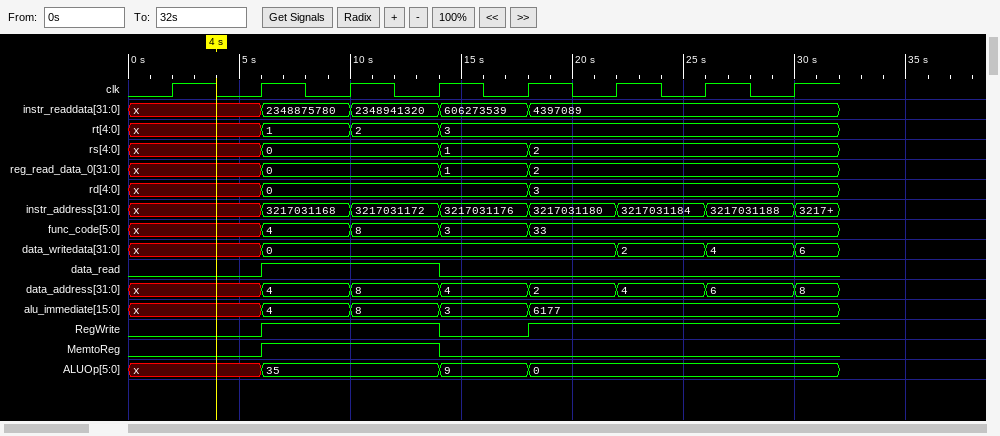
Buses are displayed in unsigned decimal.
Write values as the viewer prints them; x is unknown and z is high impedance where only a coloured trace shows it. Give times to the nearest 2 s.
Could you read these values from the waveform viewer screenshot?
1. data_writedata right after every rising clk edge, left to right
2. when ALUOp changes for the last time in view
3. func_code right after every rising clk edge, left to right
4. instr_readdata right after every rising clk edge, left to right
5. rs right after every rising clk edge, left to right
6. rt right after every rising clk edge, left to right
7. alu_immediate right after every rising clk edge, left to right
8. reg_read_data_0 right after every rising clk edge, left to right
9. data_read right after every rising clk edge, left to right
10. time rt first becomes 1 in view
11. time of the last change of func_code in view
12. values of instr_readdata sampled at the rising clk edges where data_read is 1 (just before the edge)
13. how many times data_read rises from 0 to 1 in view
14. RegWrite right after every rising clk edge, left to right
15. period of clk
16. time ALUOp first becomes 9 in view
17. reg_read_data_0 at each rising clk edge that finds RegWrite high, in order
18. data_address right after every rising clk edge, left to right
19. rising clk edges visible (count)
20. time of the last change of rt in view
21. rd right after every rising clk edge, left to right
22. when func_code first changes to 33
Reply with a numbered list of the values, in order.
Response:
1. x, 0, 0, 0, 0, 2, 4, 6
2. 18 s
3. x, 4, 8, 3, 33, 33, 33, 33
4. x, 2348875780, 2348941320, 606273539, 4397089, 4397089, 4397089, 4397089
5. x, 0, 0, 1, 2, 2, 2, 2
6. x, 1, 2, 3, 3, 3, 3, 3
7. x, 4, 8, 3, 6177, 6177, 6177, 6177
8. x, 0, 0, 1, 2, 2, 2, 2
9. 0 1 1 0 0 0 0 0
10. 6 s
11. 18 s
12. 2348875780, 2348941320
13. 1
14. 0 1 1 0 1 1 1 1
15. 4 s
16. 14 s
17. 0, 0, 2, 2, 2
18. x, 4, 8, 4, 2, 4, 6, 8
19. 8
20. 14 s
21. x, 0, 0, 0, 3, 3, 3, 3
22. 18 s
